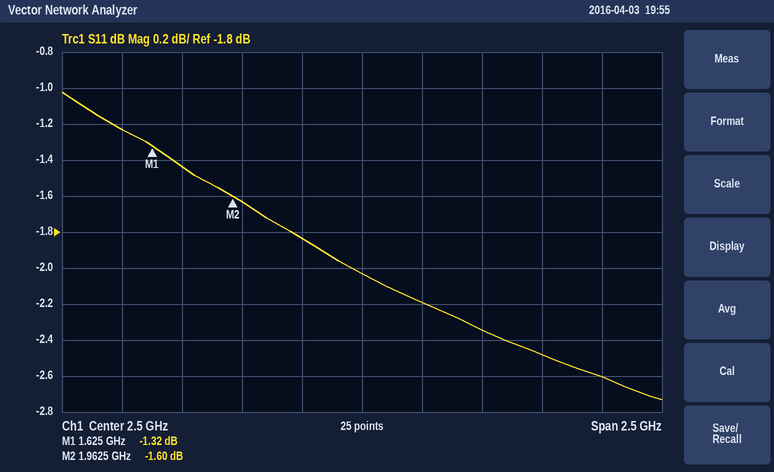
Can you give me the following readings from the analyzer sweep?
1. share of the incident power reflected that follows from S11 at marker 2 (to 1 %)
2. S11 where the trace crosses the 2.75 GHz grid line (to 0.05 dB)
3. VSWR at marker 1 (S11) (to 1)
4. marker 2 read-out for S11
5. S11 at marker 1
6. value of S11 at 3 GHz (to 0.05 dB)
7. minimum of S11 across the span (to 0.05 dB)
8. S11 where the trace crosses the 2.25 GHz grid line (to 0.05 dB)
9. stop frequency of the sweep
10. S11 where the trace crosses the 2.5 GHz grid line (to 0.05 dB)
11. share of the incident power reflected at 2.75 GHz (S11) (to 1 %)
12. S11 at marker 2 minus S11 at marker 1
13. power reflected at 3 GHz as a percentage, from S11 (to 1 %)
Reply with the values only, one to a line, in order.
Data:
69 %
-2.20 dB
13
-1.60 dB
-1.32 dB
-2.35 dB
-2.75 dB
-1.85 dB
3.75 GHz
-2.05 dB
60 %
-0.28 dB
58 %
